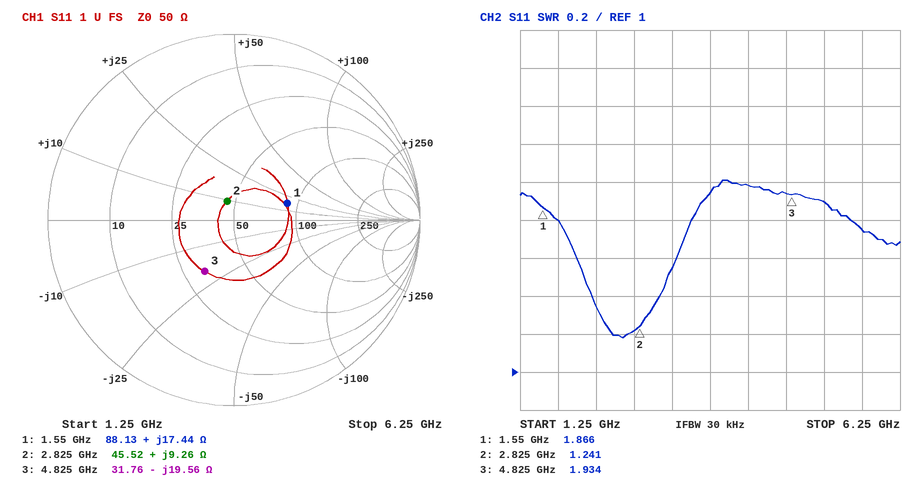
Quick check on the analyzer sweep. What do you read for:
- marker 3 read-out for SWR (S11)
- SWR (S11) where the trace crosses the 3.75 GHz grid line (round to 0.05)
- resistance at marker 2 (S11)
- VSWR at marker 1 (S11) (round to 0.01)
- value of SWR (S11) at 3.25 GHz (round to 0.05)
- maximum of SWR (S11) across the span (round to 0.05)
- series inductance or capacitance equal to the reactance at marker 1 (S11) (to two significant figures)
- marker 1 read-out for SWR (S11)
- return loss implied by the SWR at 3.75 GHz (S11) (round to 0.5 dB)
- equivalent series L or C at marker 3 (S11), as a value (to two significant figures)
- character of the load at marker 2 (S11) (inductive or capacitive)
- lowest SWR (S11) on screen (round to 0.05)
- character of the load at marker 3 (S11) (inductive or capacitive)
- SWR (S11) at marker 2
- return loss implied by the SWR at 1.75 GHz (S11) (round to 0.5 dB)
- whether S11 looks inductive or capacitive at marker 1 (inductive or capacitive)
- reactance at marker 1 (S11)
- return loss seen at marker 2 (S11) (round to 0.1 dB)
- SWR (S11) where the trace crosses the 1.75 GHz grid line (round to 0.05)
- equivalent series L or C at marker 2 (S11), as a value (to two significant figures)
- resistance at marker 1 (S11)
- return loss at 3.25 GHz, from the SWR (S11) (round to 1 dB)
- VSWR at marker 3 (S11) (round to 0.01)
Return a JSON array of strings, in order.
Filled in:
["1.934", "1.95", "45.52 Ω", "1.86", "1.55", "2.00", "1.8 nH", "1.866", "10.0 dB", "1.7 pF", "inductive", "1.20", "capacitive", "1.241", "11.0 dB", "inductive", "+17.44 Ω", "19.4 dB", "1.80", "520 pH", "88.13 Ω", "13 dB", "1.93"]
